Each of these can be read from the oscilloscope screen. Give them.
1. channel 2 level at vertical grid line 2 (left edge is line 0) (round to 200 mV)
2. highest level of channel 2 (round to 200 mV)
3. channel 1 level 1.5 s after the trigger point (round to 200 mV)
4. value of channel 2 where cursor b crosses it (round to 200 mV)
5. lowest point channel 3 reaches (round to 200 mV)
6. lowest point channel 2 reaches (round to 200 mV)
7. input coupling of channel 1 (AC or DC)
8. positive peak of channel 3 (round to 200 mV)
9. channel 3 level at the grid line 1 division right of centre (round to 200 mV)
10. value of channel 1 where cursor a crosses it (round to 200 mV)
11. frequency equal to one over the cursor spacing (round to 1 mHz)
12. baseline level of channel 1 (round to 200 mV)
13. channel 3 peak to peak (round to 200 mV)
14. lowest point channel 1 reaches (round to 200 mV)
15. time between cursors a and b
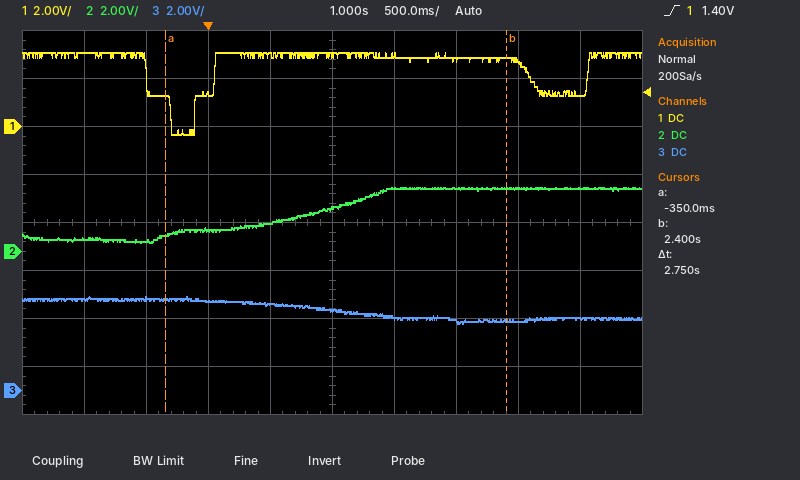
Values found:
400 mV
2.6 V
3.0 V
2.6 V
2.8 V
400 mV
DC
4.0 V
3.0 V
1.2 V
364 mHz
3.0 V
1.2 V
-400 mV
2.75 s
